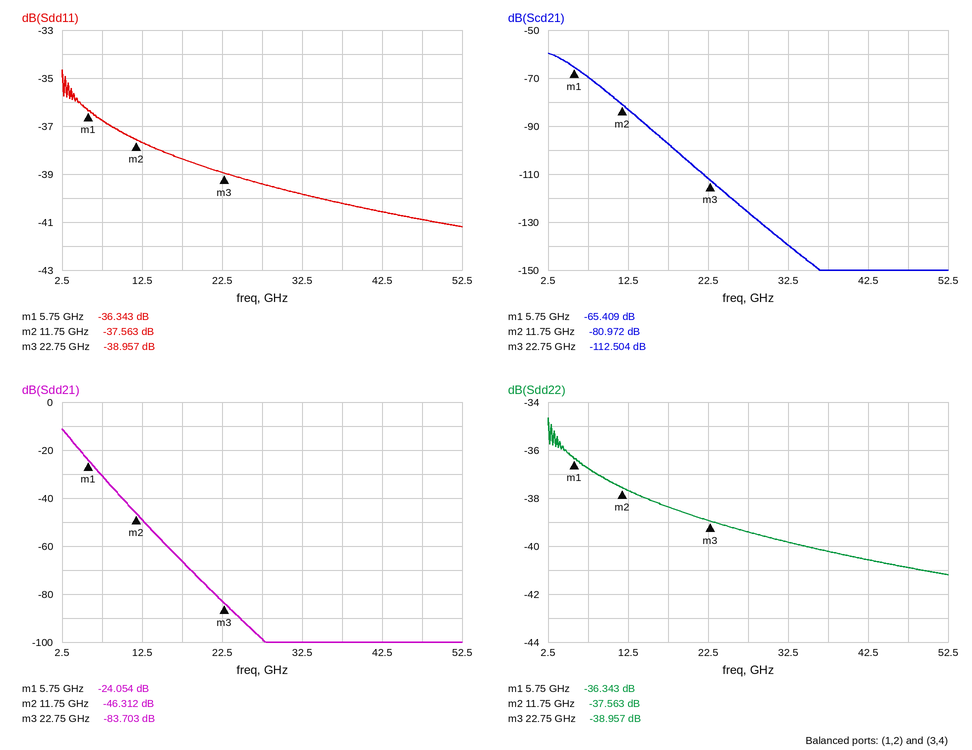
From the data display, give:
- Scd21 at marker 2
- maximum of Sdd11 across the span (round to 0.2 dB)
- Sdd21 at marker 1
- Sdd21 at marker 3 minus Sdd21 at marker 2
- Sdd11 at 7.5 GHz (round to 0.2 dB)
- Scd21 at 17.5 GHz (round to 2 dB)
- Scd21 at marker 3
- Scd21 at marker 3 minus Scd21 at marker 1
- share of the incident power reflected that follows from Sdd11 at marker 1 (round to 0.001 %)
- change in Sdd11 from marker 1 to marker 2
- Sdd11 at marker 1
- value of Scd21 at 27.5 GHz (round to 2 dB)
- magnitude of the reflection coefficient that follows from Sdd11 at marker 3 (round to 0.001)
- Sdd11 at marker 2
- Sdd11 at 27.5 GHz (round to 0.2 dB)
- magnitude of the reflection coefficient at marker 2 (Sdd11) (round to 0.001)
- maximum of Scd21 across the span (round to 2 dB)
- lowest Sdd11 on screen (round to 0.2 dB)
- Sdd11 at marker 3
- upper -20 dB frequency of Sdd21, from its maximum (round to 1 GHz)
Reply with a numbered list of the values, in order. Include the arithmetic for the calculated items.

1. -80.972 dB
2. -34.6 dB
3. -24.054 dB
4. -83.703 − (-46.312) = -37.391 dB
5. -36.8 dB
6. -98 dB
7. -112.504 dB
8. -112.504 − (-65.409) = -47.095 dB
9. 10^(-36.343/10) ≈ 0.023 %
10. -37.563 − (-36.343) = -1.220 dB
11. -36.343 dB
12. -126 dB
13. 10^(-38.957/20) ≈ 0.011
14. -37.563 dB
15. -39.4 dB
16. 10^(-37.563/20) ≈ 0.013
17. -60 dB
18. -41.2 dB
19. -38.957 dB
20. 8 GHz
